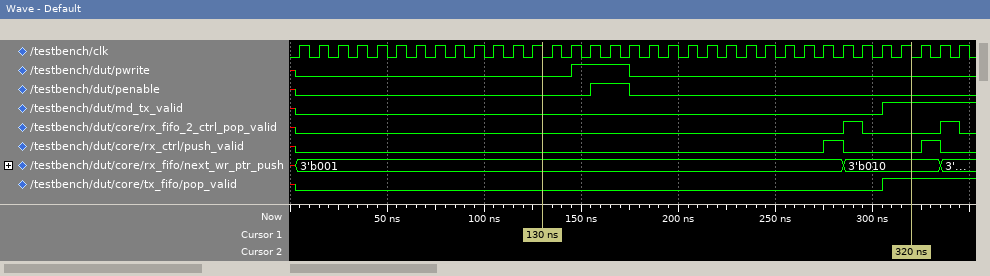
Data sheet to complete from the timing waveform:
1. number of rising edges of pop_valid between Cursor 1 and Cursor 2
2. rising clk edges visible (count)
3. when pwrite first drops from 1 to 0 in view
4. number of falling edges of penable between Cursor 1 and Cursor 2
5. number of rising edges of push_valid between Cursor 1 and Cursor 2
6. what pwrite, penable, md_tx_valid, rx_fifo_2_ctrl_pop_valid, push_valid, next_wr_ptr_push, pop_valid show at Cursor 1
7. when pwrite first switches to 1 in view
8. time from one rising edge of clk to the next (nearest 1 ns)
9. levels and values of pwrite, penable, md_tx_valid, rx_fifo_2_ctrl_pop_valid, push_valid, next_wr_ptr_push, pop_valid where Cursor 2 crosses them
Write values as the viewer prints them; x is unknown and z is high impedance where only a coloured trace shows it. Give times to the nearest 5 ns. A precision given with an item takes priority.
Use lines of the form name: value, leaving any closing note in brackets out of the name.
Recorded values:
number of rising edges of pop_valid between Cursor 1 and Cursor 2: 1
rising clk edges visible: 35
when pwrite first drops from 1 to 0 in view: 175 ns
number of falling edges of penable between Cursor 1 and Cursor 2: 1
number of rising edges of push_valid between Cursor 1 and Cursor 2: 1
what pwrite, penable, md_tx_valid, rx_fifo_2_ctrl_pop_valid, push_valid, next_wr_ptr_push, pop_valid show at Cursor 1: pwrite=0, penable=0, md_tx_valid=0, rx_fifo_2_ctrl_pop_valid=0, push_valid=0, next_wr_ptr_push=3'b001, pop_valid=0
when pwrite first switches to 1 in view: 145 ns
time from one rising edge of clk to the next: 10 ns
levels and values of pwrite, penable, md_tx_valid, rx_fifo_2_ctrl_pop_valid, push_valid, next_wr_ptr_push, pop_valid where Cursor 2 crosses them: pwrite=0, penable=0, md_tx_valid=1, rx_fifo_2_ctrl_pop_valid=0, push_valid=0, next_wr_ptr_push=3'b010, pop_valid=1
